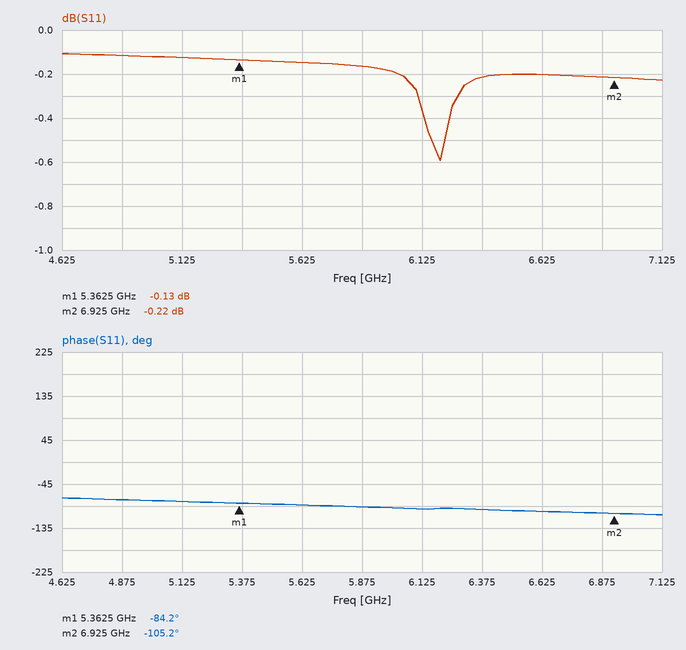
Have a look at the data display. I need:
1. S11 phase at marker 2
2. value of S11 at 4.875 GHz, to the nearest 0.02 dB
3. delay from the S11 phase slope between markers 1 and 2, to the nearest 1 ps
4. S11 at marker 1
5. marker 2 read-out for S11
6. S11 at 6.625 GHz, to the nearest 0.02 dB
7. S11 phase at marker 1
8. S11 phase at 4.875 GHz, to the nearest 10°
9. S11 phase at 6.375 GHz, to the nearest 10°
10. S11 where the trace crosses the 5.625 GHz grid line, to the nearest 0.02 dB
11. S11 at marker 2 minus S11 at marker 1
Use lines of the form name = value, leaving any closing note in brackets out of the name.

S11 phase at marker 2 = -105.2°
value of S11 at 4.875 GHz, to the nearest 0.02 dB = -0.12 dB
delay from the S11 phase slope between markers 1 and 2, to the nearest 1 ps = 37 ps
S11 at marker 1 = -0.13 dB
marker 2 read-out for S11 = -0.22 dB
S11 at 6.625 GHz, to the nearest 0.02 dB = -0.20 dB
S11 phase at marker 1 = -84.2°
S11 phase at 4.875 GHz, to the nearest 10° = -80°
S11 phase at 6.375 GHz, to the nearest 10° = -100°
S11 where the trace crosses the 5.625 GHz grid line, to the nearest 0.02 dB = -0.14 dB
S11 at marker 2 minus S11 at marker 1 = -0.09 dB
